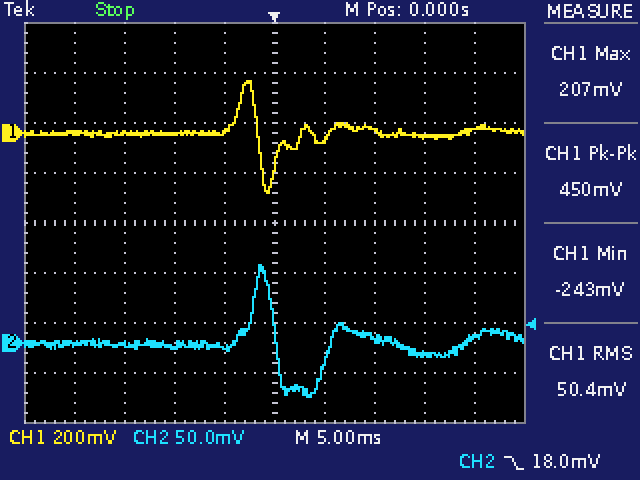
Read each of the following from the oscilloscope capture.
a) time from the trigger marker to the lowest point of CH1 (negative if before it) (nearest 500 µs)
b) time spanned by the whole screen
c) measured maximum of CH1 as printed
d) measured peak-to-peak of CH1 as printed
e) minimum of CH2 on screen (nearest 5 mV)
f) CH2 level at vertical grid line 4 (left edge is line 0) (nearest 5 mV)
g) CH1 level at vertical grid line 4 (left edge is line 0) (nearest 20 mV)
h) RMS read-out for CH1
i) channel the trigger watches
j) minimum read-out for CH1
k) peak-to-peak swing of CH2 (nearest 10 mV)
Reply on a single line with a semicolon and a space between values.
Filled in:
-500 µs; 50 ms; 207 mV; 450 mV; -55 mV; -5 mV; 0 mV; 50.4 mV; CH2; -243 mV; 130 mV
